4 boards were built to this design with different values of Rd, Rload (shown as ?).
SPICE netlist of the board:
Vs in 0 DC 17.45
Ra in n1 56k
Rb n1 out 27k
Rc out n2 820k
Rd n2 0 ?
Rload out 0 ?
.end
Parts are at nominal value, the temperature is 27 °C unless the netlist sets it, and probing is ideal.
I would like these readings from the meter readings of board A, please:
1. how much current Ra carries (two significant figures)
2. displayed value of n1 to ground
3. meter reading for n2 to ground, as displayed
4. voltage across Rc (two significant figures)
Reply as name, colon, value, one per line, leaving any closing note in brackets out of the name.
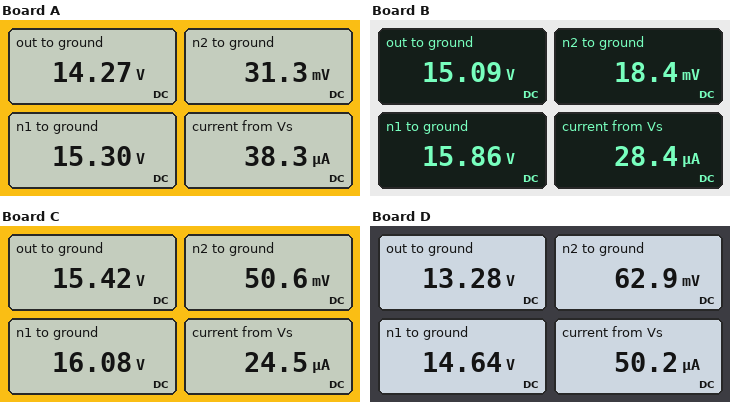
how much current Ra carries: 38 µA
displayed value of n1 to ground: 15.30 V
meter reading for n2 to ground, as displayed: 31.3 mV
voltage across Rc: 14 V
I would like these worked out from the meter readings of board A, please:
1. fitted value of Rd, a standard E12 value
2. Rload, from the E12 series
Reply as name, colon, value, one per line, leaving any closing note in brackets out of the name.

fitted value of Rd, a standard E12 value: 1.8 kΩ
Rload, from the E12 series: 680 kΩ
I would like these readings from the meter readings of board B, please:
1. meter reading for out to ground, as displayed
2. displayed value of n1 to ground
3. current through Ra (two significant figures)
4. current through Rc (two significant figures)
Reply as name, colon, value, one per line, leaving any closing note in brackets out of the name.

meter reading for out to ground, as displayed: 15.09 V
displayed value of n1 to ground: 15.86 V
current through Ra: 28 µA
current through Rc: 18 µA
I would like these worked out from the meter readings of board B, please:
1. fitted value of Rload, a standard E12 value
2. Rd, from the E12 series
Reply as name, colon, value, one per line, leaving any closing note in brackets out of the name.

fitted value of Rload, a standard E12 value: 1.5 MΩ
Rd, from the E12 series: 1 kΩ
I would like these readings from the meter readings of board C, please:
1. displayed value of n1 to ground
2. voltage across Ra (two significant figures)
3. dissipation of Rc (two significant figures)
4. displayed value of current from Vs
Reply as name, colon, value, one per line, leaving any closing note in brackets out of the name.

displayed value of n1 to ground: 16.08 V
voltage across Ra: 1.4 V
dissipation of Rc: 290 µW
displayed value of current from Vs: 24.5 µA
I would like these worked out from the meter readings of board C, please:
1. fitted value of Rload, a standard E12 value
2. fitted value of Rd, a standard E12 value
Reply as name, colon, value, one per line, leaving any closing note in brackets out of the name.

fitted value of Rload, a standard E12 value: 2.7 MΩ
fitted value of Rd, a standard E12 value: 2.7 kΩ
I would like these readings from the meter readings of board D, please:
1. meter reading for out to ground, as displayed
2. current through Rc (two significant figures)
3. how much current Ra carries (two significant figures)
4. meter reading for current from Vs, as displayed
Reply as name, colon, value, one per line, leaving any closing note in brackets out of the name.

meter reading for out to ground, as displayed: 13.28 V
current through Rc: 16 µA
how much current Ra carries: 50 µA
meter reading for current from Vs, as displayed: 50.2 µA
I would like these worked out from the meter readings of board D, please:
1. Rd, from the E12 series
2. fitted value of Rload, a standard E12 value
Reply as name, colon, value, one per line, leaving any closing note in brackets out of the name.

Rd, from the E12 series: 3.9 kΩ
fitted value of Rload, a standard E12 value: 390 kΩ
